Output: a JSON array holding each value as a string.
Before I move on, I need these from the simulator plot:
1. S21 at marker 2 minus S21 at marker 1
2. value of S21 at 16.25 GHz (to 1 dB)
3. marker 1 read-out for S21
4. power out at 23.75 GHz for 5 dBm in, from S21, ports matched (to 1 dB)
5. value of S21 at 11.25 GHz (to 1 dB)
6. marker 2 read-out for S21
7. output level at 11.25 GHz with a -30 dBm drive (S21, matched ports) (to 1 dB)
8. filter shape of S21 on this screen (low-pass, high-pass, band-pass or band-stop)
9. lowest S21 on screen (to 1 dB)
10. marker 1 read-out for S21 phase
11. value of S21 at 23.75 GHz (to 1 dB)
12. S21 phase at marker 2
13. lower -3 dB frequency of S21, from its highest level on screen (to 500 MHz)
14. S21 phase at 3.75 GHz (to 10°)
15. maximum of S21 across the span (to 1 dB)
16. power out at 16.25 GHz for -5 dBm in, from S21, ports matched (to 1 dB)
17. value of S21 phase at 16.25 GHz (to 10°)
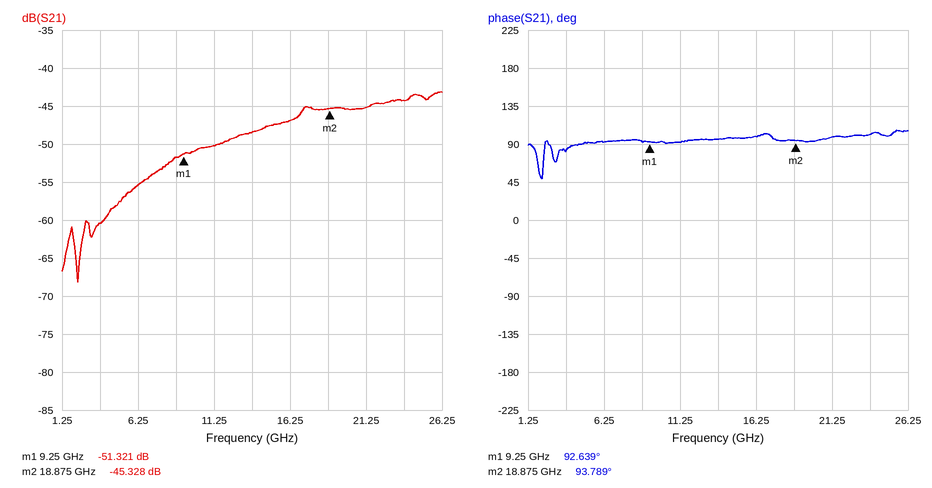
["5.993 dB", "-47 dB", "-51.321 dB", "-39 dBm", "-50 dB", "-45.328 dB", "-80 dBm", "high-pass", "-68 dB", "92.639°", "-44 dB", "93.789°", "17.0 GHz", "80°", "-43 dB", "-52 dBm", "100°"]
